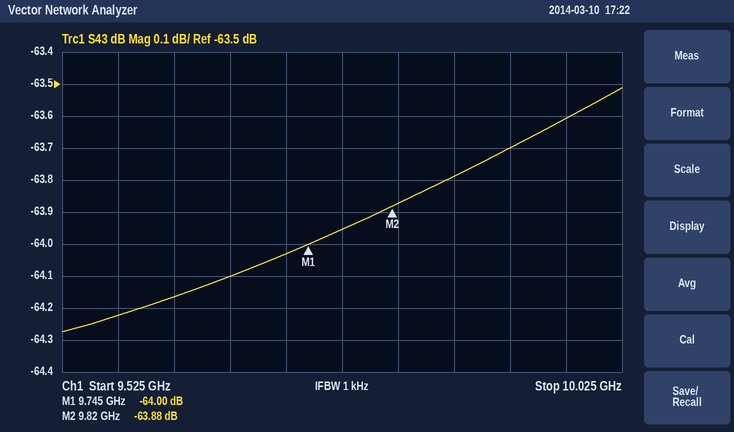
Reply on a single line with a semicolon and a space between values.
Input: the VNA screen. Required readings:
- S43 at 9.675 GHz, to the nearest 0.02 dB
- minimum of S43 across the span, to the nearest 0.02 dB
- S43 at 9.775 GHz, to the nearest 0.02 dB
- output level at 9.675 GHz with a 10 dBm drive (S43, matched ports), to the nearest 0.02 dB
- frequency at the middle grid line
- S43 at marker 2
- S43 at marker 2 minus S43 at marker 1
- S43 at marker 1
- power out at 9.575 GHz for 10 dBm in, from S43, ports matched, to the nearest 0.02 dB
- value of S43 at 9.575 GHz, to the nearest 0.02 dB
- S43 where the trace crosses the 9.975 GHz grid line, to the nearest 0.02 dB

-64.10 dB; -64.28 dB; -63.96 dB; -54.10 dBm; 9.775 GHz; -63.88 dB; 0.12 dB; -64.00 dB; -54.22 dBm; -64.22 dB; -63.60 dB
